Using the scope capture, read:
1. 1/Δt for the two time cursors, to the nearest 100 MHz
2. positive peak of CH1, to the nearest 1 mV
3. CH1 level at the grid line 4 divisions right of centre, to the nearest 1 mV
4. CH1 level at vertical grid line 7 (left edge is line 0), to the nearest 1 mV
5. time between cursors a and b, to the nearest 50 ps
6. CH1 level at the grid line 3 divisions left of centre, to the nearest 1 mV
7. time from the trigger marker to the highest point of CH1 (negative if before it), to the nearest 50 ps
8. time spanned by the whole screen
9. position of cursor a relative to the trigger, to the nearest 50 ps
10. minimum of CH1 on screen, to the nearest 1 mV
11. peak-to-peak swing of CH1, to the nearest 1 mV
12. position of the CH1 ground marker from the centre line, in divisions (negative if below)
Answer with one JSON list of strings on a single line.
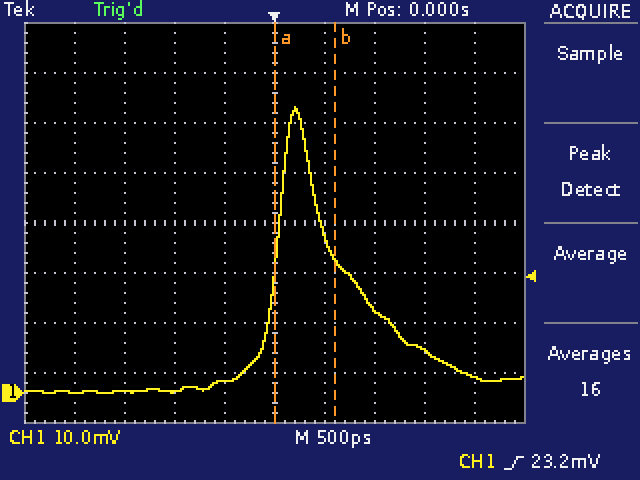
["1.7 GHz", "57 mV", "3 mV", "17 mV", "600 ps", "0 mV", "+200 ps", "5 ns", "0 ps", "0 mV", "57 mV", "-3.4 div"]
